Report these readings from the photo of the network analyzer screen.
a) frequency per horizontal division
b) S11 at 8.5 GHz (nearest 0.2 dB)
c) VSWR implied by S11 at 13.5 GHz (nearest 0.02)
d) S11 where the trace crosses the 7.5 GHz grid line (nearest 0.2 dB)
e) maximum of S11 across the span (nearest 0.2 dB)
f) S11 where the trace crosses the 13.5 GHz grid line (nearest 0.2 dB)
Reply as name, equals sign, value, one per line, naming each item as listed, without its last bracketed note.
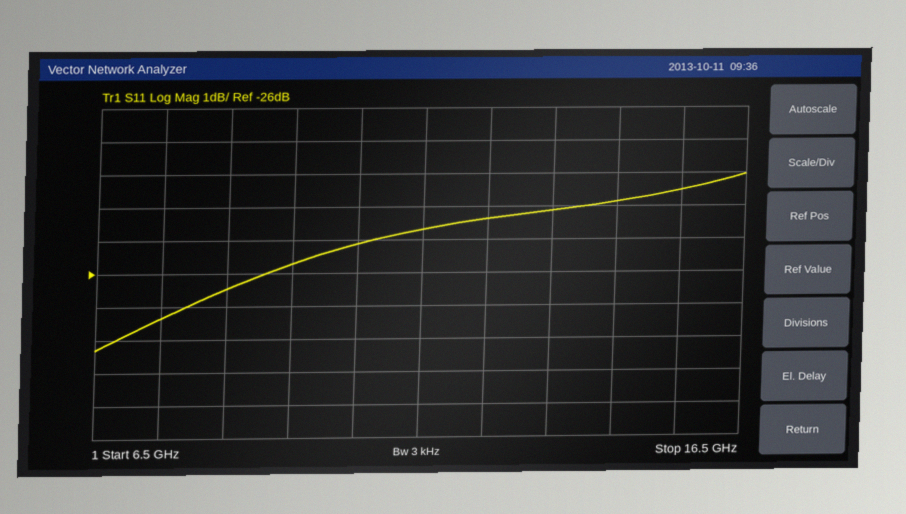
frequency per horizontal division = 1 GHz
S11 at 8.5 GHz = -26.4 dB
VSWR implied by S11 at 13.5 GHz = 1.14
S11 where the trace crosses the 7.5 GHz grid line = -27.4 dB
maximum of S11 across the span = -23.0 dB
S11 where the trace crosses the 13.5 GHz grid line = -24.2 dB
